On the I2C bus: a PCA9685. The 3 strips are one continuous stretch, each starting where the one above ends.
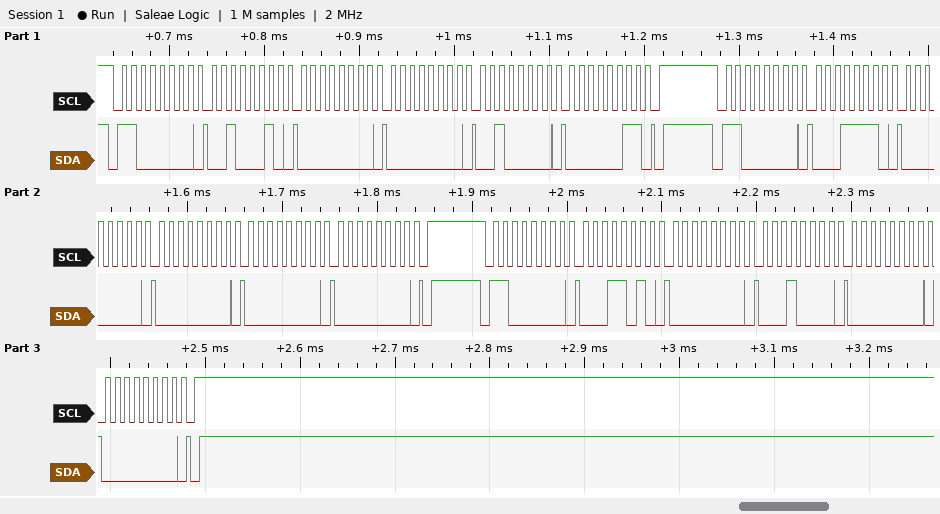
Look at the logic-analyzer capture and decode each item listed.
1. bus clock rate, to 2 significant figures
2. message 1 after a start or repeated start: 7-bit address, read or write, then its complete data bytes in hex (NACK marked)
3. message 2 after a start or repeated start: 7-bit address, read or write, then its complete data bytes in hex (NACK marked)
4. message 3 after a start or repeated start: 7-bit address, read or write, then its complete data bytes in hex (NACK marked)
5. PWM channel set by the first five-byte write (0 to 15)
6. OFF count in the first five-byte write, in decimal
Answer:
100 kHz
0x60 write: 22 00 00 20 03
0x60 write: 1E 00 00 00 00
0x60 write: 1A 00 10 00 00
7
800
